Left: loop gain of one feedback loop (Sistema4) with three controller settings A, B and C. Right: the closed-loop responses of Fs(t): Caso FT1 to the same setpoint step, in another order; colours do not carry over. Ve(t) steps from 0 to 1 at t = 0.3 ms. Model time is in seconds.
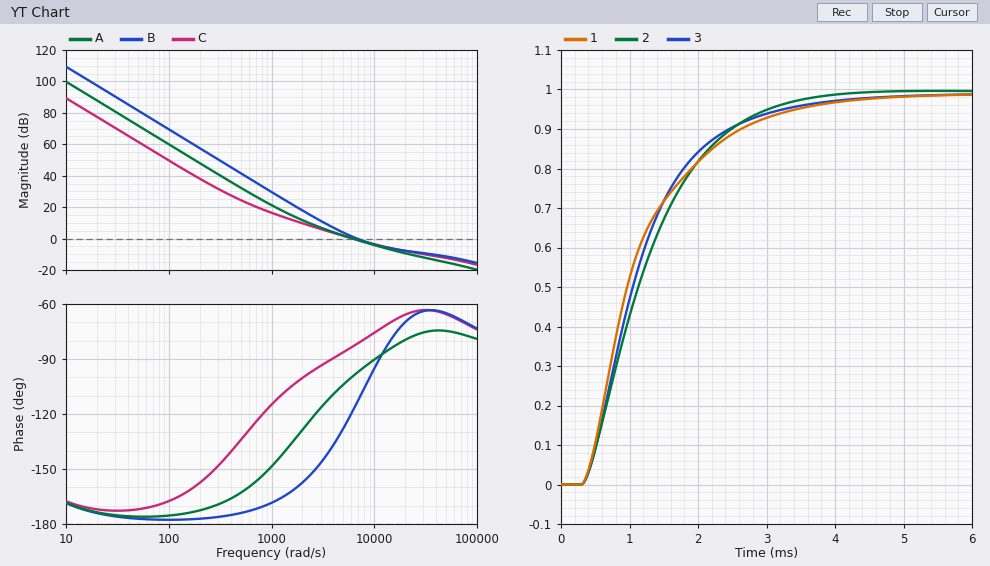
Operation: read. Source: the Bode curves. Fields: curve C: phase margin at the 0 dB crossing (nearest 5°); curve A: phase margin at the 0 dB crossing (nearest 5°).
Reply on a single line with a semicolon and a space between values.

95°; 80°
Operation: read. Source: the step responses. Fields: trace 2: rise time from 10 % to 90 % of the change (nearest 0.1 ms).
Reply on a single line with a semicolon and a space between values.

1.9 ms
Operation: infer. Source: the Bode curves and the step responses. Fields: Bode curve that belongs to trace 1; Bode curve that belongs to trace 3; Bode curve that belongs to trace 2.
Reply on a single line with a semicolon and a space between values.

B; A; C
